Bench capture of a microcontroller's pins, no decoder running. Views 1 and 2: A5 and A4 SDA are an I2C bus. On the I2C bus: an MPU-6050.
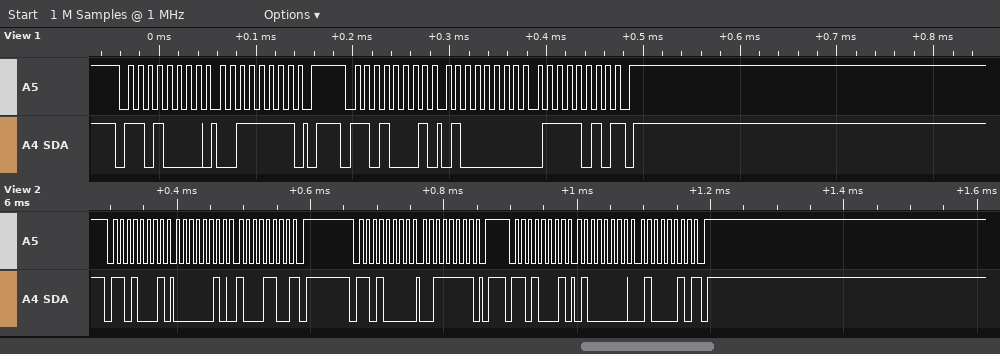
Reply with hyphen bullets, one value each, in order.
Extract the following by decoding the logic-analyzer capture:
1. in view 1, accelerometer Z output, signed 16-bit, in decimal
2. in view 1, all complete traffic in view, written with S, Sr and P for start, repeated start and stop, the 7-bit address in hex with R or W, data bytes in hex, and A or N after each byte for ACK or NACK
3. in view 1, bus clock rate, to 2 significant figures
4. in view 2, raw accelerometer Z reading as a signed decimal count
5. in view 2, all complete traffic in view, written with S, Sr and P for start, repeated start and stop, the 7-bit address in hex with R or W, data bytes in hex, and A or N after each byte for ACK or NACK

- 16506
- S 68W A 3F A P S 68R A 40 A 7A N P
- 100 kHz
- 16450
- S 68R A 02 A 8C N P S 68W A 3F A P S 68R A 40 A 42 N P
